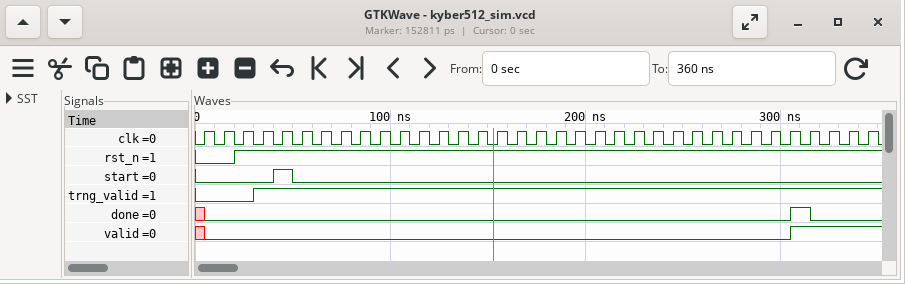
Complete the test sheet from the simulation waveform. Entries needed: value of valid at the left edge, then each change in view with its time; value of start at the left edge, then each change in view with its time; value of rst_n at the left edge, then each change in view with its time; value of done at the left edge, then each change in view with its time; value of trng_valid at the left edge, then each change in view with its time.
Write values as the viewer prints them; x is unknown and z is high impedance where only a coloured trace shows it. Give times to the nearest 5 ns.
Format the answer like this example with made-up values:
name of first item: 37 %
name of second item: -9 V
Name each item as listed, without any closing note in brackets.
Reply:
value of valid at the left edge, then each change in view with its time: x, 0 at 5 ns, 1 at 305 ns
value of start at the left edge, then each change in view with its time: 0, 1 at 40 ns, 0 at 50 ns
value of rst_n at the left edge, then each change in view with its time: 0, 1 at 20 ns
value of done at the left edge, then each change in view with its time: x, 0 at 5 ns, 1 at 305 ns, 0 at 315 ns
value of trng_valid at the left edge, then each change in view with its time: 0, 1 at 30 ns
